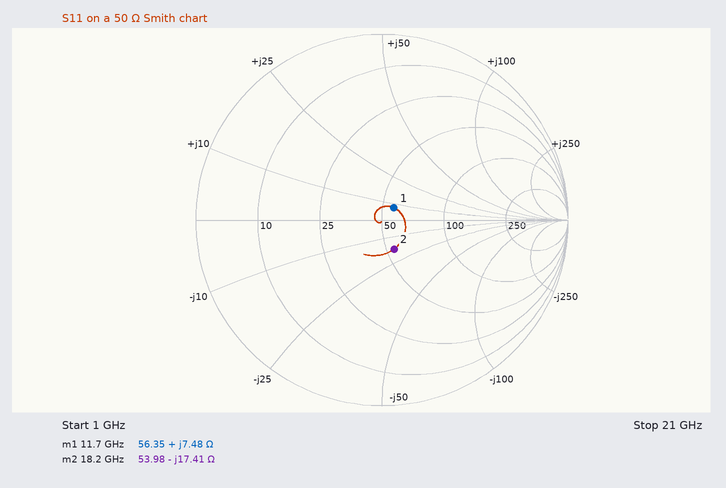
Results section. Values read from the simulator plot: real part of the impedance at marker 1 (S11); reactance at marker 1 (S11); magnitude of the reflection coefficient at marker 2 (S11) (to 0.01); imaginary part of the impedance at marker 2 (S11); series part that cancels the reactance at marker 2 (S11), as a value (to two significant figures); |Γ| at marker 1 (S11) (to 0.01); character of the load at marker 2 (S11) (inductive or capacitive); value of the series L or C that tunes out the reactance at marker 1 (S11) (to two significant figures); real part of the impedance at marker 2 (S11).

56.35 Ω
+7.48 Ω
0.17
-17.41 Ω
150 pH
0.09
capacitive
1.8 pF
53.98 Ω
